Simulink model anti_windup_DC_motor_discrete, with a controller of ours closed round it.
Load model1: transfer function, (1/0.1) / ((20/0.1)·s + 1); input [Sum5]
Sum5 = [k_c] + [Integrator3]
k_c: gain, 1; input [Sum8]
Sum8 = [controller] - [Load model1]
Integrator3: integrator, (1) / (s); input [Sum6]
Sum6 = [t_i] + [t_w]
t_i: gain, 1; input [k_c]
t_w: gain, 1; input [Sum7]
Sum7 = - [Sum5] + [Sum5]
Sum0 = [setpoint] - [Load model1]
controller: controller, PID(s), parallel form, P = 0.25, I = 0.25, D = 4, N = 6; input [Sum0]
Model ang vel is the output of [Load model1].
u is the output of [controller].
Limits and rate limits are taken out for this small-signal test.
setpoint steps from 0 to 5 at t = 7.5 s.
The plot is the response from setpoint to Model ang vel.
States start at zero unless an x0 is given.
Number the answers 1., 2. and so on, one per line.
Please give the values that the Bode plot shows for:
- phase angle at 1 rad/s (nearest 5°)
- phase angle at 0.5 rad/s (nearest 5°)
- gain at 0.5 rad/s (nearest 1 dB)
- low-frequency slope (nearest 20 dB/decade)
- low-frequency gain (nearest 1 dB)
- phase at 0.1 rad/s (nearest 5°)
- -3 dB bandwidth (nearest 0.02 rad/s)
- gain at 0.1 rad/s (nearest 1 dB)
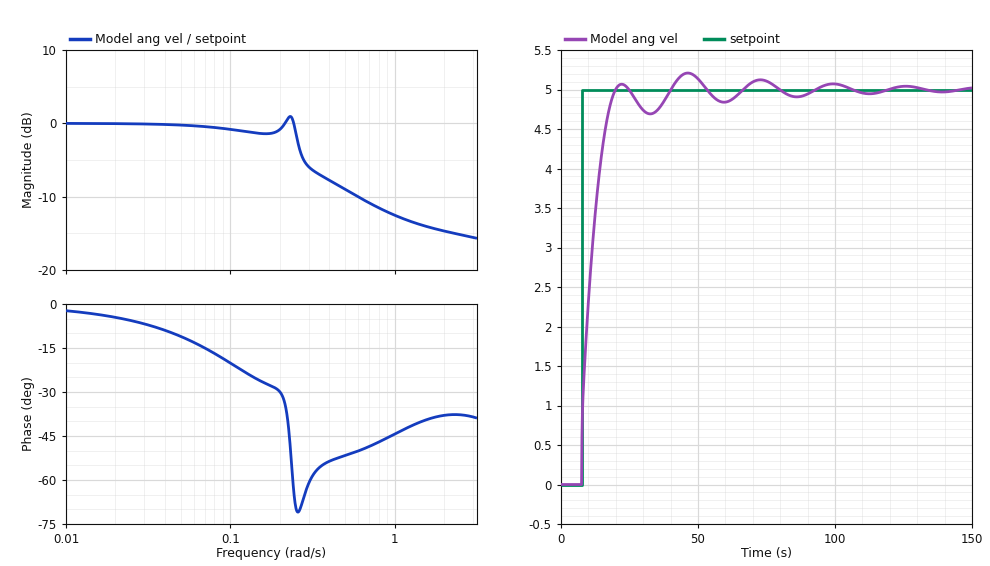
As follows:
1. -45°
2. -50°
3. -9 dB
4. 0 dB/decade
5. 0 dB
6. -20°
7. 0.26 rad/s
8. -1 dB
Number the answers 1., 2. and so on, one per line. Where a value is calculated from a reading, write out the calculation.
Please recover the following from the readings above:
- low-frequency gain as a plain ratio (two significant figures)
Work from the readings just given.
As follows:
1. 10^(0 / 20) = 1.0
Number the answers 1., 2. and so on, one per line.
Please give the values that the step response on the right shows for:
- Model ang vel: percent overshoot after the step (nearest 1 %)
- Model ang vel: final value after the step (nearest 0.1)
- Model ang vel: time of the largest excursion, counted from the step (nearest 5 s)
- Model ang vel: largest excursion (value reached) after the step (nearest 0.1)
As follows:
1. 4 %
2. 5.0
3. 40 s
4. 5.2
